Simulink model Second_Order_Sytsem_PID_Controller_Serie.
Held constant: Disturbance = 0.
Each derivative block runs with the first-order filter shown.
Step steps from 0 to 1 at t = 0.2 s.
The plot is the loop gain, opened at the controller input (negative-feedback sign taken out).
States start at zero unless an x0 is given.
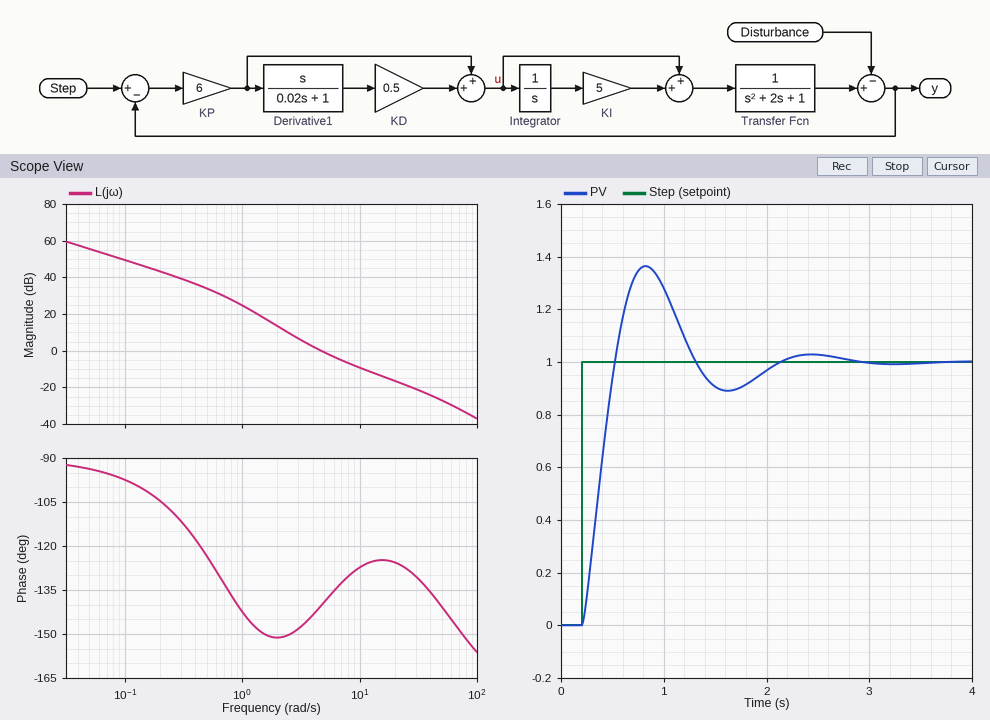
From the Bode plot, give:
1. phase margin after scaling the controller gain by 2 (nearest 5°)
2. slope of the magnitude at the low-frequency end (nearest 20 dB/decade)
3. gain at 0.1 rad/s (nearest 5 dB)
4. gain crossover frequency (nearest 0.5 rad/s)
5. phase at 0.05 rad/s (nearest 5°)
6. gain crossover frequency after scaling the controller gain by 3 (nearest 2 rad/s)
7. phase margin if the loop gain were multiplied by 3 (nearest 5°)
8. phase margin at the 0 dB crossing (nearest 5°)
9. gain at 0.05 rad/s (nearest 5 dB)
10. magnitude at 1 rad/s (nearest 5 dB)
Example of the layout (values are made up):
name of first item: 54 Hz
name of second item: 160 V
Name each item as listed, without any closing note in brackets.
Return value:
phase margin after scaling the controller gain by 2: 50°
slope of the magnitude at the low-frequency end: -20 dB/decade
gain at 0.1 rad/s: 50 dB
gain crossover frequency: 4.5 rad/s
phase at 0.05 rad/s: -95°
gain crossover frequency after scaling the controller gain by 3: 10 rad/s
phase margin if the loop gain were multiplied by 3: 55°
phase margin at the 0 dB crossing: 40°
gain at 0.05 rad/s: 55 dB
magnitude at 1 rad/s: 25 dB
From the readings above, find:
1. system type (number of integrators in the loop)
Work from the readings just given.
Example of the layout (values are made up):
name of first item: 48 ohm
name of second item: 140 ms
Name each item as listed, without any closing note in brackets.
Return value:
system type: 1
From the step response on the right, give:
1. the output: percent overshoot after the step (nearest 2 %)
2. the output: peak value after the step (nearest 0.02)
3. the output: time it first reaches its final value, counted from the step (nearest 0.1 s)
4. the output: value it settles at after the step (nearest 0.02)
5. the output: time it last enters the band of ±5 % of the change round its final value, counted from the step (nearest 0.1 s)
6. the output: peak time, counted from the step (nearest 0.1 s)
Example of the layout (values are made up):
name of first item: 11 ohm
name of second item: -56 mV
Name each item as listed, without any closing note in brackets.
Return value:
the output: percent overshoot after the step: 36 %
the output: peak value after the step: 1.36
the output: time it first reaches its final value, counted from the step: 0.3 s
the output: value it settles at after the step: 1.00
the output: time it last enters the band of ±5 % of the change round its final value, counted from the step: 1.7 s
the output: peak time, counted from the step: 0.6 s
